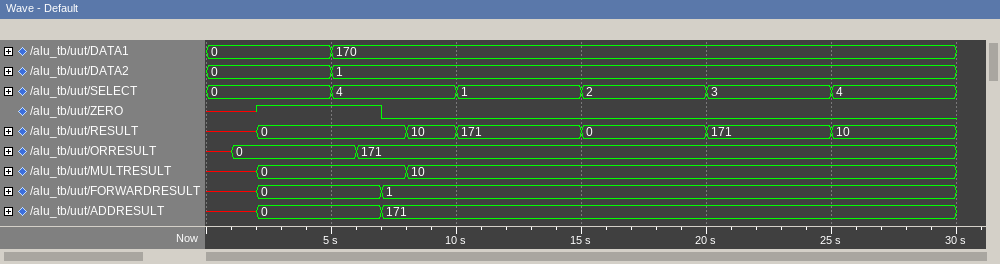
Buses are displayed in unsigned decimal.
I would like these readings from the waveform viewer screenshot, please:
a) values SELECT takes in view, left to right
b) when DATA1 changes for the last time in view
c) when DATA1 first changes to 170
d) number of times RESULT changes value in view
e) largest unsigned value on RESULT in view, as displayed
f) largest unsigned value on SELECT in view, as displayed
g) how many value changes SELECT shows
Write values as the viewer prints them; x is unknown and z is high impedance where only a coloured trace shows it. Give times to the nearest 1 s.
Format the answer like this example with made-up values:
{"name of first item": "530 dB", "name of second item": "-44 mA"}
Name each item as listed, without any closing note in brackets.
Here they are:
{"values SELECT takes in view, left to right": "0, 4, 1, 2, 3, 4", "when DATA1 changes for the last time in view": "5 s", "when DATA1 first changes to 170": "5 s", "number of times RESULT changes value in view": "6", "largest unsigned value on RESULT in view, as displayed": "171", "largest unsigned value on SELECT in view, as displayed": "4", "how many value changes SELECT shows": "5"}
